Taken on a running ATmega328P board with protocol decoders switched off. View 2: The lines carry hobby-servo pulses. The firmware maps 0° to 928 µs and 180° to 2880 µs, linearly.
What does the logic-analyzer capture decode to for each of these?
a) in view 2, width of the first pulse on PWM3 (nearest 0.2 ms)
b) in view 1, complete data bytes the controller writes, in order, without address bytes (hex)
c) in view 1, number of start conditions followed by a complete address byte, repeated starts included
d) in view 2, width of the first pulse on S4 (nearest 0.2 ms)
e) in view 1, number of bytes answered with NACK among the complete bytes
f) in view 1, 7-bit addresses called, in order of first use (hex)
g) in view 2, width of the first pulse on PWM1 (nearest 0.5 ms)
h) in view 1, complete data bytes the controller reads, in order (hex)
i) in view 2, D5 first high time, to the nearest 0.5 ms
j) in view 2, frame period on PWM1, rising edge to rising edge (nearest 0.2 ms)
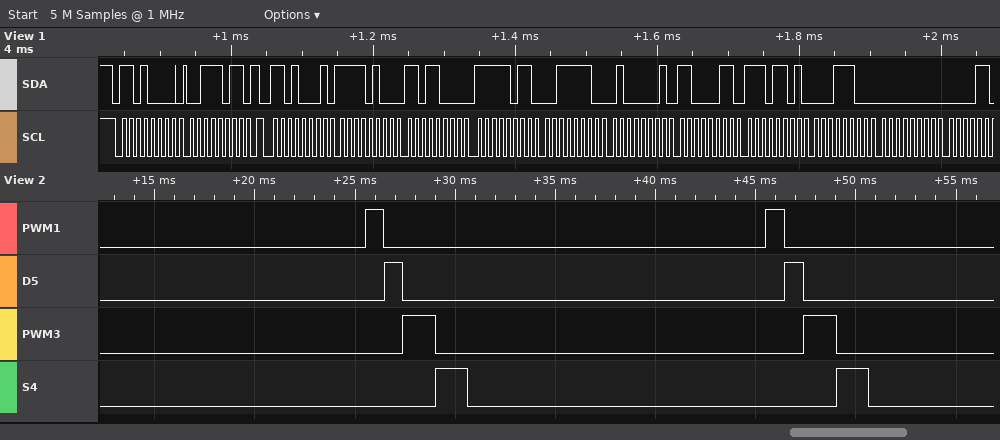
1.6 ms
3B
2
1.6 ms
0
0x68
1.0 ms
F4 D8 FB 3E 41 C3 ED 1C 00
1.0 ms
20.0 ms
